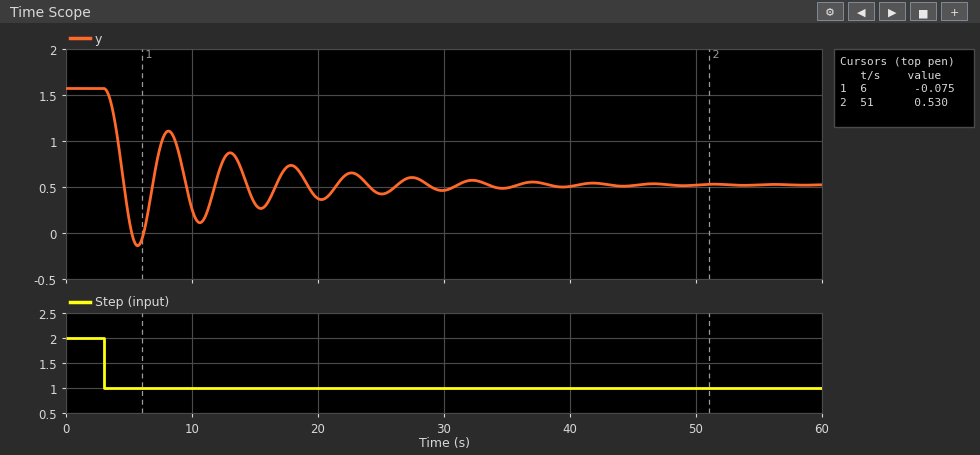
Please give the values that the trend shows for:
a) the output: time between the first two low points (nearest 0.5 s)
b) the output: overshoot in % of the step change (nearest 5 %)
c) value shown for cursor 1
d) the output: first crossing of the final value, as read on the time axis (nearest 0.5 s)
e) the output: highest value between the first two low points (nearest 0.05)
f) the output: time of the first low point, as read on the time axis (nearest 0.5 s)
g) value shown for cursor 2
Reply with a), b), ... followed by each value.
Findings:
a) 5.0 s
b) 65 %
c) -0.075
d) 4.5 s
e) 1.10
f) 5.5 s
g) 0.530
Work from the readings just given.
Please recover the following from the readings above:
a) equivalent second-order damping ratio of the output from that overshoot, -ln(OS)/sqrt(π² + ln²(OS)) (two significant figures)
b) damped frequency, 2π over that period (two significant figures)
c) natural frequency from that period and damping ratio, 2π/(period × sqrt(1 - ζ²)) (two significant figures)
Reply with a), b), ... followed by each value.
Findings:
a) 0.14
b) 1.3 rad/s
c) 1.3 rad/s
